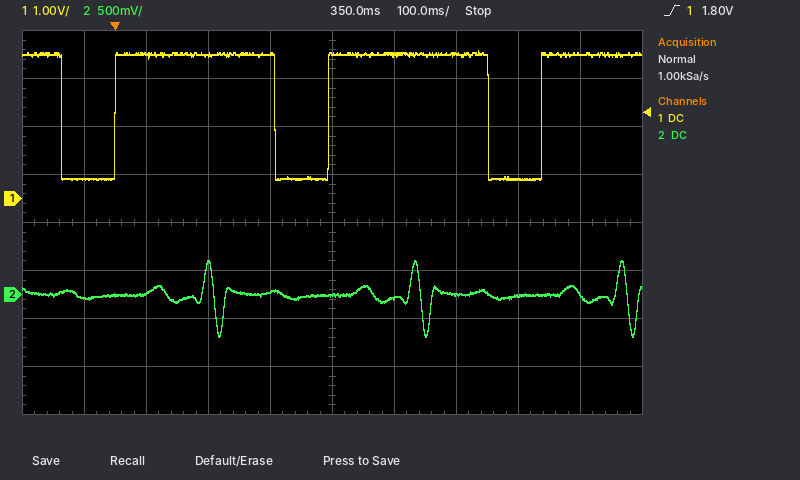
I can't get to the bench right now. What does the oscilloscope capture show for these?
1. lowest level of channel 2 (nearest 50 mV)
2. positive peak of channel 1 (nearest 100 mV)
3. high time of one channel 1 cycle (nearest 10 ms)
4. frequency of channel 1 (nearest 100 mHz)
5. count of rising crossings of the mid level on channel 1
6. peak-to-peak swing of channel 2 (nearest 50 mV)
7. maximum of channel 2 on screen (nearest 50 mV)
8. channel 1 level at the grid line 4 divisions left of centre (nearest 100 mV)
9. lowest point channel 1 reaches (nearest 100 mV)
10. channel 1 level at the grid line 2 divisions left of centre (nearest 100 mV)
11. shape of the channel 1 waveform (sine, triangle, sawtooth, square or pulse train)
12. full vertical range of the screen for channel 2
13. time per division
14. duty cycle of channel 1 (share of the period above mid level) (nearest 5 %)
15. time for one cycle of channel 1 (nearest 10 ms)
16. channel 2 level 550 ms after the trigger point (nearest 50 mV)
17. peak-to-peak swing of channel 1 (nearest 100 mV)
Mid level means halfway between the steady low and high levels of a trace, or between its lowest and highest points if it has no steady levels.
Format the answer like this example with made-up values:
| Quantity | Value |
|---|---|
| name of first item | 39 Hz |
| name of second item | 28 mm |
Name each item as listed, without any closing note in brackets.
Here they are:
| Quantity | Value |
|---|---|
| lowest level of channel 2 | -450 mV |
| positive peak of channel 1 | 3.1 V |
| high time of one channel 1 cycle | 260 ms |
| frequency of channel 1 | 2.9 Hz |
| count of rising crossings of the mid level on channel 1 | 3 |
| peak-to-peak swing of channel 2 | 800 mV |
| maximum of channel 2 on screen | 350 mV |
| channel 1 level at the grid line 4 divisions left of centre | 400 mV |
| lowest point channel 1 reaches | 400 mV |
| channel 1 level at the grid line 2 divisions left of centre | 3.0 V |
| shape of the channel 1 waveform | pulse train |
| full vertical range of the screen for channel 2 | 4 V |
| time per division | 100 ms |
| duty cycle of channel 1 (share of the period above mid level) | 75 % |
| time for one cycle of channel 1 | 340 ms |
| channel 2 level 550 ms after the trigger point | 0 mV |
| peak-to-peak swing of channel 1 | 2.7 V |
